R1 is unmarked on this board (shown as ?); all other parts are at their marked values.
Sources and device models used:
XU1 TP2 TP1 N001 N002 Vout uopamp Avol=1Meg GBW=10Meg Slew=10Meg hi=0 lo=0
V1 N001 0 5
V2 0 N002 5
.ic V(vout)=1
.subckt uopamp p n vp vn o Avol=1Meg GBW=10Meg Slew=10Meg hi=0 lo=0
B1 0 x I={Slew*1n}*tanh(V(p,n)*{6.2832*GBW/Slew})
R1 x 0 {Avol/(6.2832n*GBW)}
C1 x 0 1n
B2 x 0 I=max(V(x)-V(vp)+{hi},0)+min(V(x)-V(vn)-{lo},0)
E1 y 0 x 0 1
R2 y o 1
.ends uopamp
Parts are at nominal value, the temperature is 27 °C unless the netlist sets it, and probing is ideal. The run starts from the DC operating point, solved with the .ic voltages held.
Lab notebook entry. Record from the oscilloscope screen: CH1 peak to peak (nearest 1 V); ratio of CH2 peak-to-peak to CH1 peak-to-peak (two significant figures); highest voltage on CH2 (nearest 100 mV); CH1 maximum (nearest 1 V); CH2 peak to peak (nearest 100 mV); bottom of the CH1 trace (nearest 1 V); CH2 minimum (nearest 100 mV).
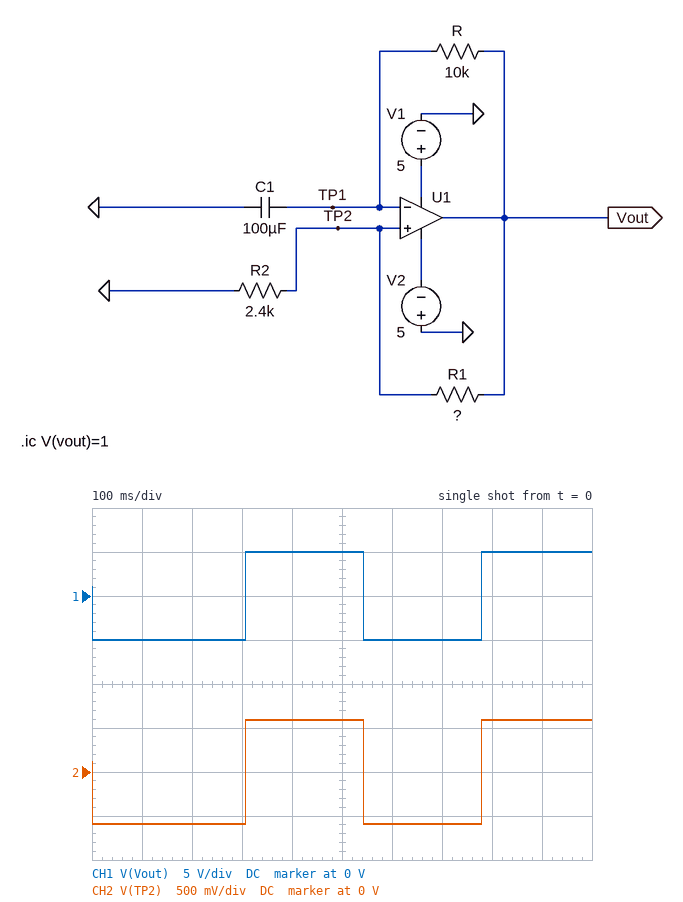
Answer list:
10 V
0.12
600 mV
5 V
1.2 V
-5 V
-600 mV
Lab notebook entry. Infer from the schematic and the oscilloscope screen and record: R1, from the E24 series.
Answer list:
18 kΩ
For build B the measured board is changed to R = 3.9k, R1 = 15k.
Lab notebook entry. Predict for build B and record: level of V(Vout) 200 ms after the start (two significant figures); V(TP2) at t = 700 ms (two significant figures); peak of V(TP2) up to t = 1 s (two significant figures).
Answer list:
5.0 V
-690 mV
690 mV
